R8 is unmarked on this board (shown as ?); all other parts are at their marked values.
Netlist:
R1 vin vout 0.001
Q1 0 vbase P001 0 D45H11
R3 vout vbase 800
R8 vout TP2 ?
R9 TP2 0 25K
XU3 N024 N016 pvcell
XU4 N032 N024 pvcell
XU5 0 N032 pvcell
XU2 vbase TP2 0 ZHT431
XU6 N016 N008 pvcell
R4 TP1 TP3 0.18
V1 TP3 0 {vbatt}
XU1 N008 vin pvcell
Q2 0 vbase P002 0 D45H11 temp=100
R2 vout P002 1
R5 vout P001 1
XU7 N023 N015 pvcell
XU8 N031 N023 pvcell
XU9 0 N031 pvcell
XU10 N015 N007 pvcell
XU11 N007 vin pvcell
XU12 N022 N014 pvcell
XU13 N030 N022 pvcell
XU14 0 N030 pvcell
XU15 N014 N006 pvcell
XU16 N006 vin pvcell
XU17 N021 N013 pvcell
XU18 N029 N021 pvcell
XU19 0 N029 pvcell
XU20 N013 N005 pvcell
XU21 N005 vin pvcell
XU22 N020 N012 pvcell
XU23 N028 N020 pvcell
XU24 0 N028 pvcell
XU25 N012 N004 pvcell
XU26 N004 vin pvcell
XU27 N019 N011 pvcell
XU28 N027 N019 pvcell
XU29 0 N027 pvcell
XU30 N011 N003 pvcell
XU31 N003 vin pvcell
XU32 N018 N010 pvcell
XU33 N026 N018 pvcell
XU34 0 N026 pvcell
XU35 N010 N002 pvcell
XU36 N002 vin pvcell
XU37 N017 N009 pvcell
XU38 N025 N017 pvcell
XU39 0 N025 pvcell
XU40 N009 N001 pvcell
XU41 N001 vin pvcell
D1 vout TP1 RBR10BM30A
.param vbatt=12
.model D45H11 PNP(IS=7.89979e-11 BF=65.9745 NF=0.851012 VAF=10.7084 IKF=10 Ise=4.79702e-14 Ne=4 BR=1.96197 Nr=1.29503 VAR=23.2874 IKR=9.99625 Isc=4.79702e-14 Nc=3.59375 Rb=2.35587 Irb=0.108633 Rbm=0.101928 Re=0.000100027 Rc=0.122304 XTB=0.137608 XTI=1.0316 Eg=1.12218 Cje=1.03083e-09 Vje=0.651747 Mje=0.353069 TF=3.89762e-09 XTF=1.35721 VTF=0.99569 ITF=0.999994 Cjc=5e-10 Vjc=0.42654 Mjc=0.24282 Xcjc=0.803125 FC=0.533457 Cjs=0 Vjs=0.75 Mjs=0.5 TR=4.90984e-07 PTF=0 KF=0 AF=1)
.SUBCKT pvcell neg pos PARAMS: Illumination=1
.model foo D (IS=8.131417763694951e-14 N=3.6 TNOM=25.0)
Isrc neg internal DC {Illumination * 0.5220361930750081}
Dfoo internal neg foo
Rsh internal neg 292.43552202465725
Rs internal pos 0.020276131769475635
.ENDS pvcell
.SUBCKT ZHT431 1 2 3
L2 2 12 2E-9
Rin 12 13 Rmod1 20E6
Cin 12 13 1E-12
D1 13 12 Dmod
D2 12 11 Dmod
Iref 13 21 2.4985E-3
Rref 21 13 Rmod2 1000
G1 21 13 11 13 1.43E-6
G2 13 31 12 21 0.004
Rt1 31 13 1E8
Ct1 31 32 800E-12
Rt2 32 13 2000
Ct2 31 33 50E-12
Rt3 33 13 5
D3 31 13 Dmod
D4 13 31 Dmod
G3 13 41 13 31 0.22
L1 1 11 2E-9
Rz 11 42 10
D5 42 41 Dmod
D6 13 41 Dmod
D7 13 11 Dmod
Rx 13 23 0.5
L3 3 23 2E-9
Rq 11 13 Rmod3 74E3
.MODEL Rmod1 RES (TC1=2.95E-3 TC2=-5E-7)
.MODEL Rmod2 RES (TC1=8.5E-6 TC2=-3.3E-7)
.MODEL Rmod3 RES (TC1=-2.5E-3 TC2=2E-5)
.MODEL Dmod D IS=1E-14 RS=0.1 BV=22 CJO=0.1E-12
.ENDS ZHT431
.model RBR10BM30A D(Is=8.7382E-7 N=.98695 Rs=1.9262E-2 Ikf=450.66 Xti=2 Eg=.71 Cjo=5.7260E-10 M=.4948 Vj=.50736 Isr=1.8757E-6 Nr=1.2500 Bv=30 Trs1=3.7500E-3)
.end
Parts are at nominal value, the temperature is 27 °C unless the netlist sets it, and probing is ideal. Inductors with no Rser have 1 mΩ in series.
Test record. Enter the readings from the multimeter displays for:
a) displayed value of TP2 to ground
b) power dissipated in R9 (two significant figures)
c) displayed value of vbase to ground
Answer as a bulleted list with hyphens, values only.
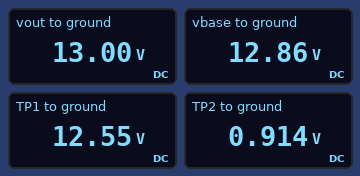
- 0.914 V
- 33 µW
- 12.86 V
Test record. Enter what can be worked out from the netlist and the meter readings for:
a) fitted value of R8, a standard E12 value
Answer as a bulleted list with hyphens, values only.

- 330 kΩ
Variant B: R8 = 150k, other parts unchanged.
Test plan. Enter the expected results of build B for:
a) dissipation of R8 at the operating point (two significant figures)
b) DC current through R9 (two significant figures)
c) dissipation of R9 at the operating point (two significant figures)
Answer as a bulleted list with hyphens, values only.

- 830 µW
- 74 µA
- 140 µW
